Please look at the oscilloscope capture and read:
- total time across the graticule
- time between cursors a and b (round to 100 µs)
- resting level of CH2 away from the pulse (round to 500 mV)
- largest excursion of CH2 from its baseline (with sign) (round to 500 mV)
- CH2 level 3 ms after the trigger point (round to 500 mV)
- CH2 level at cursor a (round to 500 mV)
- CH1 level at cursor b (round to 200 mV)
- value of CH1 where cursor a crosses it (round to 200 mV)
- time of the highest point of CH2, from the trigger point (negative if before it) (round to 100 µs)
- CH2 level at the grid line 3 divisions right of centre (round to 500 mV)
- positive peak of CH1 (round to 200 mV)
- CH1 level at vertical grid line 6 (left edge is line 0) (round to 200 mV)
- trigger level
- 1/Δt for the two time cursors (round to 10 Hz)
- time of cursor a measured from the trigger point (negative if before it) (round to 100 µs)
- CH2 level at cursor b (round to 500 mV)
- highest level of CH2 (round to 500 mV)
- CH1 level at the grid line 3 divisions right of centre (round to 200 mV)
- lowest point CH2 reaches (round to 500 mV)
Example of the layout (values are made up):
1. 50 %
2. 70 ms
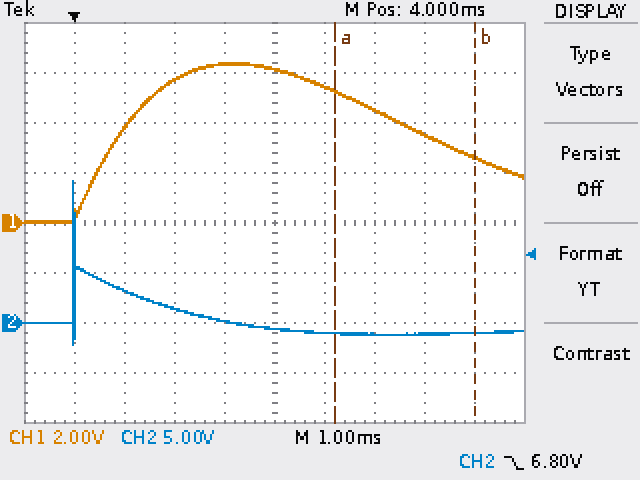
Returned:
1. 10 ms
2. 2.8 ms
3. -1.0 V
4. +15.0 V
5. 0.0 V
6. -1.0 V
7. 2.6 V
8. 5.2 V
9. 0.0 ms
10. -1.0 V
11. 6.4 V
12. 5.4 V
13. 6.80 V
14. 360 Hz
15. +5.2 ms
16. -1.0 V
17. 14.0 V
18. 3.6 V
19. -2.0 V
